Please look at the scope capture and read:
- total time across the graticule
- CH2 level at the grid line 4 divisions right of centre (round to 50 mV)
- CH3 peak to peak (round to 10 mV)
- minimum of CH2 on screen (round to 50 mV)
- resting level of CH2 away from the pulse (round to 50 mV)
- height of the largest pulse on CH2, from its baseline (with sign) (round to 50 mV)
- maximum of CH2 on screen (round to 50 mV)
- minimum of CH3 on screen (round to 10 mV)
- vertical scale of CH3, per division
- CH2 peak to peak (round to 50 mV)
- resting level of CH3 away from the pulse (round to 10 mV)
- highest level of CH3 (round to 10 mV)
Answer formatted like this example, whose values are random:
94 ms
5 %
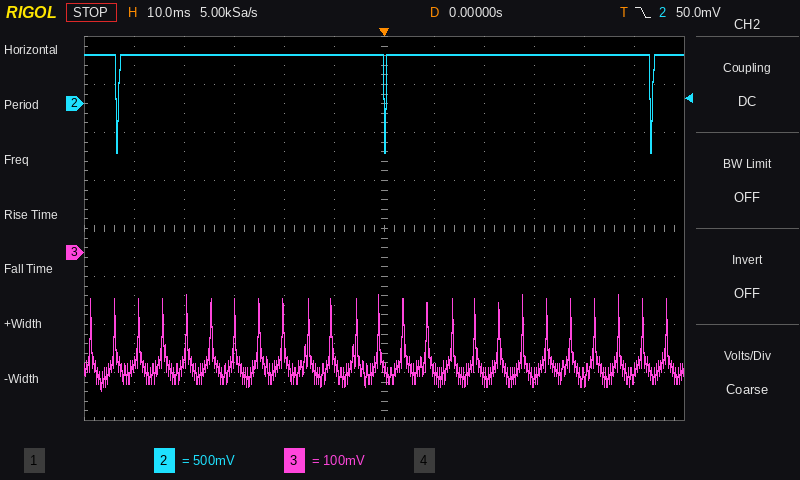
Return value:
120 ms
500 mV
200 mV
-500 mV
500 mV
-1.00 V
500 mV
-290 mV
100 mV
1.00 V
-240 mV
-90 mV
